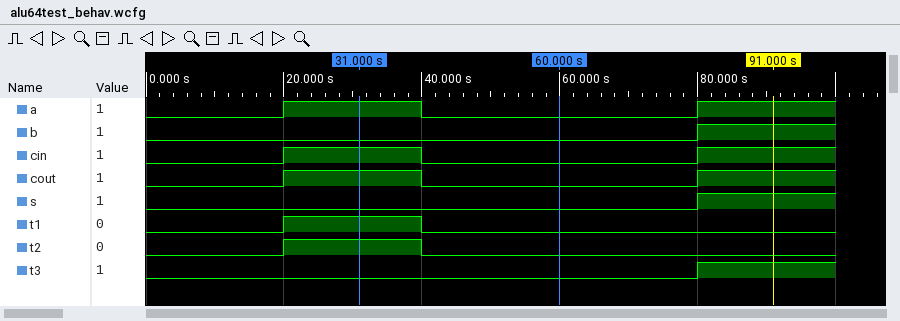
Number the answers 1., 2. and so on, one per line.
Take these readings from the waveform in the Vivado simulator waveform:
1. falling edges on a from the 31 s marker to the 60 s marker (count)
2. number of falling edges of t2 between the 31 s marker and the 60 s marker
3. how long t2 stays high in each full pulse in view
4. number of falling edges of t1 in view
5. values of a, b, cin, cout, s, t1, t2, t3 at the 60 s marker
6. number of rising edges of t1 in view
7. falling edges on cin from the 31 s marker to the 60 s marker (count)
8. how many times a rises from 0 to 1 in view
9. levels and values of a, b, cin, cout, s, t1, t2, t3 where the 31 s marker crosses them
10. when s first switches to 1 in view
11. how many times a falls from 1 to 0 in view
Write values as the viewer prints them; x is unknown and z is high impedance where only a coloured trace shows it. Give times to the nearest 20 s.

1. 1
2. 1
3. 20 s
4. 1
5. a=0, b=0, cin=0, cout=0, s=0, t1=0, t2=0, t3=0
6. 1
7. 1
8. 2
9. a=1, b=0, cin=1, cout=1, s=0, t1=1, t2=1, t3=0
10. 80 s
11. 1
